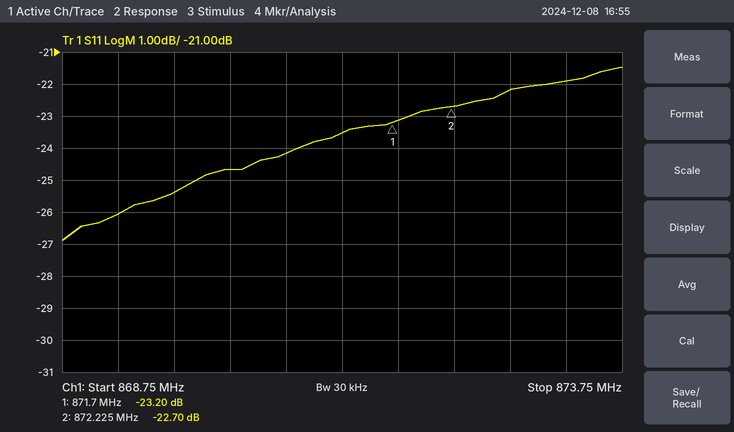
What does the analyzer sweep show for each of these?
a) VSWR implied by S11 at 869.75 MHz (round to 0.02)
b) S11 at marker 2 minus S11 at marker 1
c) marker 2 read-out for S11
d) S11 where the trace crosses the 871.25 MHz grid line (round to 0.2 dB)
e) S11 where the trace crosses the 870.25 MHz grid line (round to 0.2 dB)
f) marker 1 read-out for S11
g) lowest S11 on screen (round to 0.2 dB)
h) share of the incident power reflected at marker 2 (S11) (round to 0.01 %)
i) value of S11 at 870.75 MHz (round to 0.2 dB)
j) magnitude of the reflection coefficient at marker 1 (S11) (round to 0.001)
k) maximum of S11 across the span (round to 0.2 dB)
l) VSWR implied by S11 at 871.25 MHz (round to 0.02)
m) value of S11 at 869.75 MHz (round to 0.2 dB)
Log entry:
1.12
0.50 dB
-22.70 dB
-23.6 dB
-24.6 dB
-23.20 dB
-26.8 dB
0.54 %
-24.2 dB
0.069
-21.4 dB
1.14
-25.4 dB
